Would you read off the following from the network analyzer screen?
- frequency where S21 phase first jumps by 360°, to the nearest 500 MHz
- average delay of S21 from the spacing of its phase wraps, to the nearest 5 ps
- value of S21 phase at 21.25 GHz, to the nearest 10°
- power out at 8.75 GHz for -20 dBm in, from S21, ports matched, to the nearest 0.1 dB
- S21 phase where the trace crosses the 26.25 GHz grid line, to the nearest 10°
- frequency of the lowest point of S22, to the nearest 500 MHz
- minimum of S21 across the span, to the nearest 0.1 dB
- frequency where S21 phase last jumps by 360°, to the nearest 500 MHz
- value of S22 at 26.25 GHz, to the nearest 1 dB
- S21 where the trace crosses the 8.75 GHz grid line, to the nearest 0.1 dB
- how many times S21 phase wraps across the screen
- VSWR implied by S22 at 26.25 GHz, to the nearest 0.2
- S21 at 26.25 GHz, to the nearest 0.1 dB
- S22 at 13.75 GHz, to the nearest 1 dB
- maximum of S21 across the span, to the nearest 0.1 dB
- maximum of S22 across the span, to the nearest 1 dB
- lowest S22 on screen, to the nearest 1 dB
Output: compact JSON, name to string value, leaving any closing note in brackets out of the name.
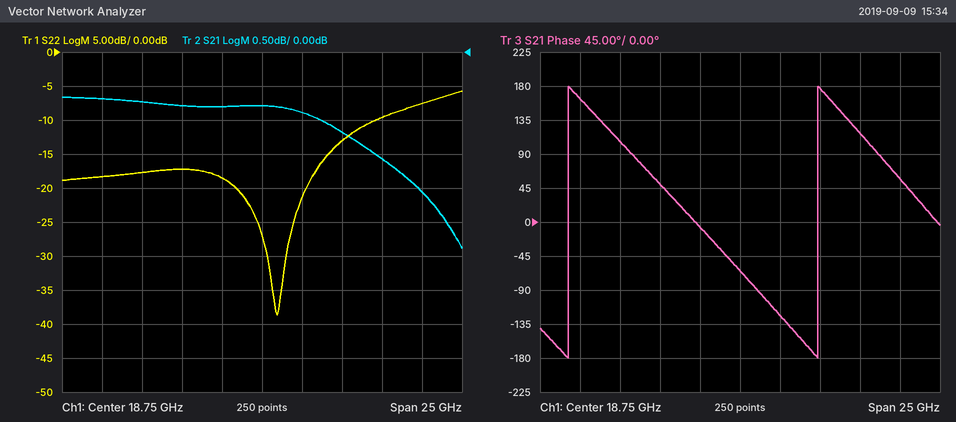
{"frequency where S21 phase first jumps by 360°, to the nearest 500 MHz": "8.0 GHz", "average delay of S21 from the spacing of its phase wraps, to the nearest 5 ps": "65 ps", "value of S21 phase at 21.25 GHz, to the nearest 10°": "-120°", "power out at 8.75 GHz for -20 dBm in, from S21, ports matched, to the nearest 0.1 dB": "-20.7 dBm", "S21 phase where the trace crosses the 26.25 GHz grid line, to the nearest 10°": "120°", "frequency of the lowest point of S22, to the nearest 500 MHz": "19.5 GHz", "minimum of S21 across the span, to the nearest 0.1 dB": "-2.9 dB", "frequency where S21 phase last jumps by 360°, to the nearest 500 MHz": "23.5 GHz", "value of S22 at 26.25 GHz, to the nearest 1 dB": "-10 dB", "S21 where the trace crosses the 8.75 GHz grid line, to the nearest 0.1 dB": "-0.7 dB", "how many times S21 phase wraps across the screen": "2", "VSWR implied by S22 at 26.25 GHz, to the nearest 0.2": "2.0", "S21 at 26.25 GHz, to the nearest 0.1 dB": "-1.6 dB", "S22 at 13.75 GHz, to the nearest 1 dB": "-17 dB", "maximum of S21 across the span, to the nearest 0.1 dB": "-0.7 dB", "maximum of S22 across the span, to the nearest 1 dB": "-6 dB", "lowest S22 on screen, to the nearest 1 dB": "-39 dB"}
